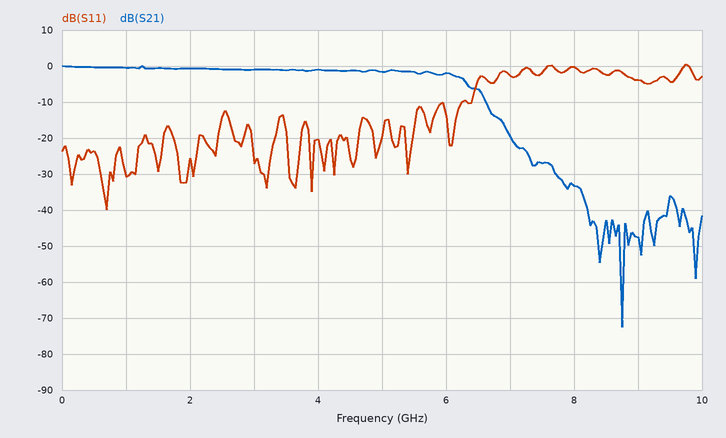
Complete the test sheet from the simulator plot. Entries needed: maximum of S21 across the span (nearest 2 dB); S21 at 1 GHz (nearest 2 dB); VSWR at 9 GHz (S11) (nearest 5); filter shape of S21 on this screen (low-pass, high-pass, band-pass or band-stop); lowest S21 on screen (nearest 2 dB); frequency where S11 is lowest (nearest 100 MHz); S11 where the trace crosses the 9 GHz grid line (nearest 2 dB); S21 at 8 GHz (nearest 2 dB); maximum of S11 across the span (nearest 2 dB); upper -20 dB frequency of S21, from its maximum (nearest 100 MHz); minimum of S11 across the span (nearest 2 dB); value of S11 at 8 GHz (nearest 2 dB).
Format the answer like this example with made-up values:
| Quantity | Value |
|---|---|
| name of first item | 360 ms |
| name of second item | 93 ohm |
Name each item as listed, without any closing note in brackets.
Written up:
| Quantity | Value |
|---|---|
| maximum of S21 across the span | 0 dB |
| S21 at 1 GHz | 0 dB |
| VSWR at 9 GHz (S11) | 5 |
| filter shape of S21 on this screen | low-pass |
| lowest S21 on screen | -72 dB |
| frequency where S11 is lowest | 700 MHz |
| S11 where the trace crosses the 9 GHz grid line | -4 dB |
| S21 at 8 GHz | -34 dB |
| maximum of S11 across the span | 0 dB |
| upper -20 dB frequency of S21, from its maximum | 7.0 GHz |
| minimum of S11 across the span | -40 dB |
| value of S11 at 8 GHz | 0 dB |
